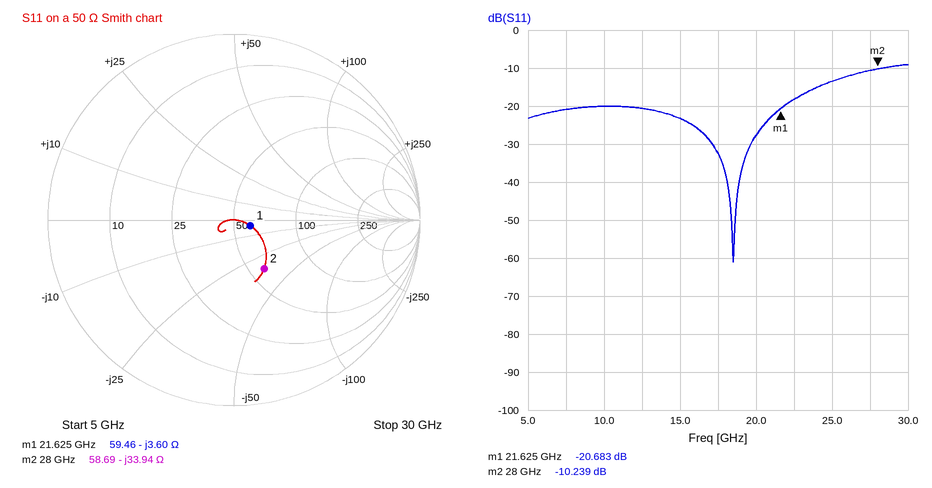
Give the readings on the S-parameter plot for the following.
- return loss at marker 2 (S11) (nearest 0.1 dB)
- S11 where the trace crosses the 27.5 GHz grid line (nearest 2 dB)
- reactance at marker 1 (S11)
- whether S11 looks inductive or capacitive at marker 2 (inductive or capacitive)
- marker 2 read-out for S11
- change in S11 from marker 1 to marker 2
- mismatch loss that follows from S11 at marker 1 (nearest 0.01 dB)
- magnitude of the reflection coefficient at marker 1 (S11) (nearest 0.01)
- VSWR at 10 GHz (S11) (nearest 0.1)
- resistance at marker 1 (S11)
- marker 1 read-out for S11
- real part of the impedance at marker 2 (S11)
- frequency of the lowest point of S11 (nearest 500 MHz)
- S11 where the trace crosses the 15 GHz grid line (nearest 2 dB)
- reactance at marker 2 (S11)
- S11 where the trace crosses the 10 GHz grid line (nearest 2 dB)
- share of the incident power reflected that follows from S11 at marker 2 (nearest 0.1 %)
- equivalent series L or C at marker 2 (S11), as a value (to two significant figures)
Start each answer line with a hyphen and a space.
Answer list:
- 10.2 dB
- -10 dB
- -3.60 Ω
- capacitive
- -10.239 dB
- 10.444 dB
- 0.04 dB
- 0.09
- 1.2
- 59.46 Ω
- -20.683 dB
- 58.69 Ω
- 18.5 GHz
- -24 dB
- -33.94 Ω
- -20 dB
- 9.5 %
- 170 fF
